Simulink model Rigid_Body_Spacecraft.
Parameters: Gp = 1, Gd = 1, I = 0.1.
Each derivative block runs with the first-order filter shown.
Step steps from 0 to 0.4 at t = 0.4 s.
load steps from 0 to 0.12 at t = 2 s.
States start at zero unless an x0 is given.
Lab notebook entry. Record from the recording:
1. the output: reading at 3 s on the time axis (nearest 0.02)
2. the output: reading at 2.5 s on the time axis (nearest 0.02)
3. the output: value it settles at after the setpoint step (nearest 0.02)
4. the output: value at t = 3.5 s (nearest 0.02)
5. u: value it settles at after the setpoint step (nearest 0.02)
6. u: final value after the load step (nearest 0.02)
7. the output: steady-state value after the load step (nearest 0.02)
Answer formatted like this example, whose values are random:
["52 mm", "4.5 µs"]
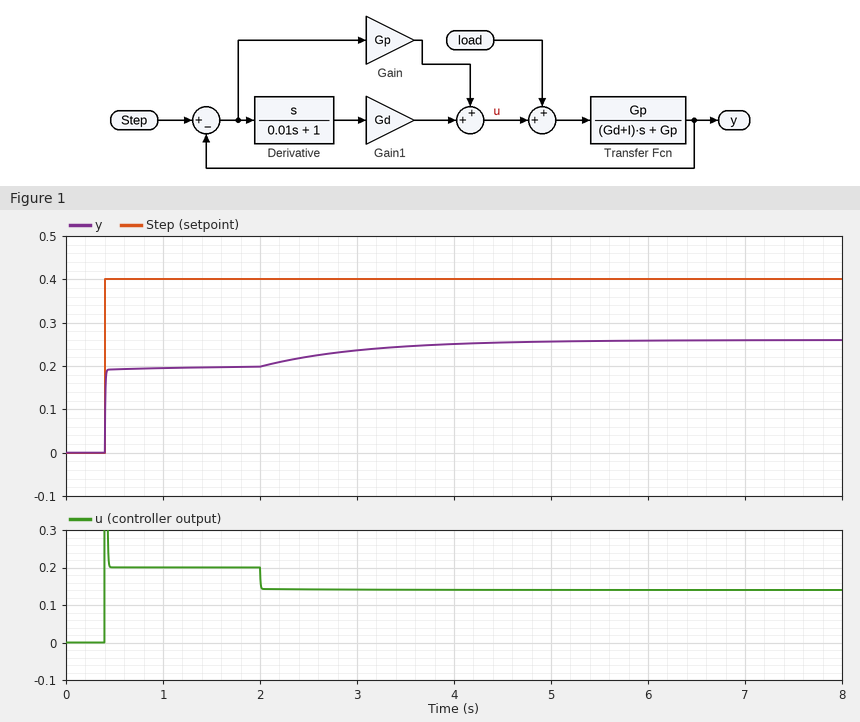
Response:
["0.24", "0.22", "0.20", "0.24", "0.20", "0.14", "0.26"]
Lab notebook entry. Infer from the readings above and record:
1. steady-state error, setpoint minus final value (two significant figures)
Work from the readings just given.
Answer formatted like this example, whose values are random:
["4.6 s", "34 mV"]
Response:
["0.20"]
